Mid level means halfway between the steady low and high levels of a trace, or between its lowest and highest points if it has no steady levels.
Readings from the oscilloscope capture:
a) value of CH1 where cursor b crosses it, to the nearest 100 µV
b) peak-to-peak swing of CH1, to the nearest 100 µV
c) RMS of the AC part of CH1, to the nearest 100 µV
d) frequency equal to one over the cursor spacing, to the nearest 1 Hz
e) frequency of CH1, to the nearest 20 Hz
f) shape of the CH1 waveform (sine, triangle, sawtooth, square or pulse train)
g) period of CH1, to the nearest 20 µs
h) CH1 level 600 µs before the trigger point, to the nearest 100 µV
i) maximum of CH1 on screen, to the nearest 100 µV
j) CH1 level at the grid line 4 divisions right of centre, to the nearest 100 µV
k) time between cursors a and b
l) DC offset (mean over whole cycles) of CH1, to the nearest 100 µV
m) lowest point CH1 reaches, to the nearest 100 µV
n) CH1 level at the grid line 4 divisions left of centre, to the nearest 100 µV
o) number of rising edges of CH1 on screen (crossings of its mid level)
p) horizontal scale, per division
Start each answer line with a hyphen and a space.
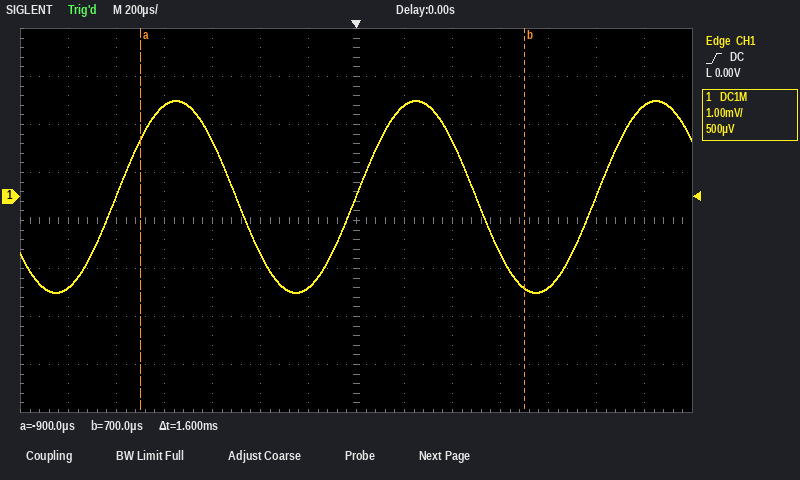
- -1.9 mV
- 4.0 mV
- 1.4 mV
- 625 Hz
- 1.00 kHz
- sine
- 1.00 ms
- 1.2 mV
- 2.0 mV
- -1.9 mV
- 1.6 ms
- 0.0 mV
- -2.0 mV
- 1.9 mV
- 3
- 200 µs
